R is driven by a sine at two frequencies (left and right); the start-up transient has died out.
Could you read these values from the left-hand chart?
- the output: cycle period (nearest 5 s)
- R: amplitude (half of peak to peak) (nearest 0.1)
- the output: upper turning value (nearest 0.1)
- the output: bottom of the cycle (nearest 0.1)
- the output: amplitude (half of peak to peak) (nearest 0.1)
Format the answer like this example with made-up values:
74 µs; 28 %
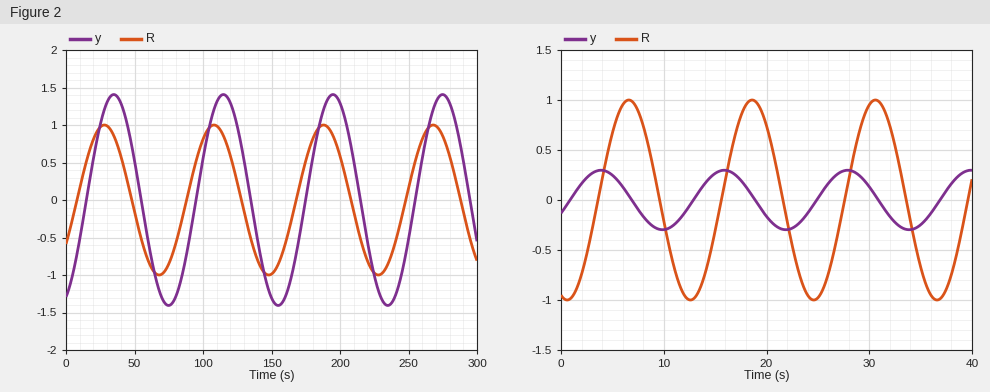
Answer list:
80 s; 1.0; 1.4; -1.4; 1.4
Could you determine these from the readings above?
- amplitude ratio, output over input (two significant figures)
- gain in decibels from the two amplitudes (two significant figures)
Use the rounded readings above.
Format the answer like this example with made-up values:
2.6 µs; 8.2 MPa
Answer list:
1.4; 2.9 dB
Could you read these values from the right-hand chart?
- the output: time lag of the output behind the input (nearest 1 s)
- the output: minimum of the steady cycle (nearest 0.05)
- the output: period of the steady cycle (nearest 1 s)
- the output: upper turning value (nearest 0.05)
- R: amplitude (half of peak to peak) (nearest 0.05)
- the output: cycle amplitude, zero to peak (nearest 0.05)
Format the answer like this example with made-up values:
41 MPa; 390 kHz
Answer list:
9 s; -0.30; 12 s; 0.30; 1.00; 0.30
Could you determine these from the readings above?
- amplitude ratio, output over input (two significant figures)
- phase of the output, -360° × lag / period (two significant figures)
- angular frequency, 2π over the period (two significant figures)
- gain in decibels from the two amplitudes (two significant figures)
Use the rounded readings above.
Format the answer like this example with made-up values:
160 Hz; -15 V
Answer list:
0.30; -270°; 0.52 rad/s; -10 dB
